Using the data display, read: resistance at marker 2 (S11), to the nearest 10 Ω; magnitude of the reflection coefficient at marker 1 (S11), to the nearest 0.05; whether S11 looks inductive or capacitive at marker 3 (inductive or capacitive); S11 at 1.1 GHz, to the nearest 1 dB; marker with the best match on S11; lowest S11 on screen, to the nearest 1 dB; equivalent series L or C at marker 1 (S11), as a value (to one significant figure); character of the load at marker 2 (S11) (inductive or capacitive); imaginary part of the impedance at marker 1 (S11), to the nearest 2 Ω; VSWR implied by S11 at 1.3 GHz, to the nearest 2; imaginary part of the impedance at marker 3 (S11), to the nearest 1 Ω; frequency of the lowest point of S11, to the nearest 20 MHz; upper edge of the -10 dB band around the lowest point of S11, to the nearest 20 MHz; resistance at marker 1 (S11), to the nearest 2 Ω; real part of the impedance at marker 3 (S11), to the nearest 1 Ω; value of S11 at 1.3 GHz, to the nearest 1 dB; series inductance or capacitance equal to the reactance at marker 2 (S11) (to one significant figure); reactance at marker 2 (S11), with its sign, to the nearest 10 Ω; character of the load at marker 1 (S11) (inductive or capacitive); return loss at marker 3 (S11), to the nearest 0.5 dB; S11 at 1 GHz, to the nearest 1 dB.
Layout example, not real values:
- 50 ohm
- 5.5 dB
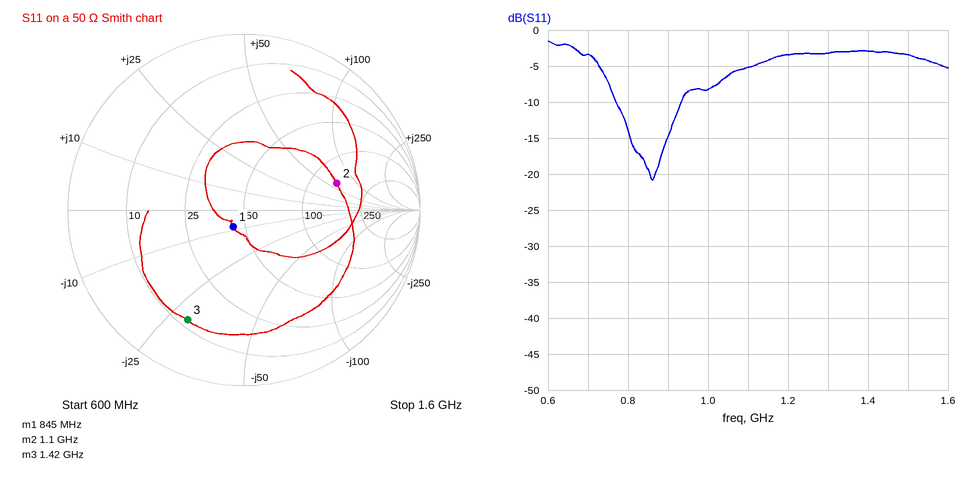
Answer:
- 140 Ω
- 0.10
- capacitive
- -5 dB
- marker 1
- -21 dB
- 20 pF
- inductive
- -8 Ω
- 6
- -29 Ω
- 860 MHz
- 940 MHz
- 44 Ω
- 12 Ω
- -3 dB
- 9 nH
- +60 Ω
- capacitive
- 3.0 dB
- -8 dB
